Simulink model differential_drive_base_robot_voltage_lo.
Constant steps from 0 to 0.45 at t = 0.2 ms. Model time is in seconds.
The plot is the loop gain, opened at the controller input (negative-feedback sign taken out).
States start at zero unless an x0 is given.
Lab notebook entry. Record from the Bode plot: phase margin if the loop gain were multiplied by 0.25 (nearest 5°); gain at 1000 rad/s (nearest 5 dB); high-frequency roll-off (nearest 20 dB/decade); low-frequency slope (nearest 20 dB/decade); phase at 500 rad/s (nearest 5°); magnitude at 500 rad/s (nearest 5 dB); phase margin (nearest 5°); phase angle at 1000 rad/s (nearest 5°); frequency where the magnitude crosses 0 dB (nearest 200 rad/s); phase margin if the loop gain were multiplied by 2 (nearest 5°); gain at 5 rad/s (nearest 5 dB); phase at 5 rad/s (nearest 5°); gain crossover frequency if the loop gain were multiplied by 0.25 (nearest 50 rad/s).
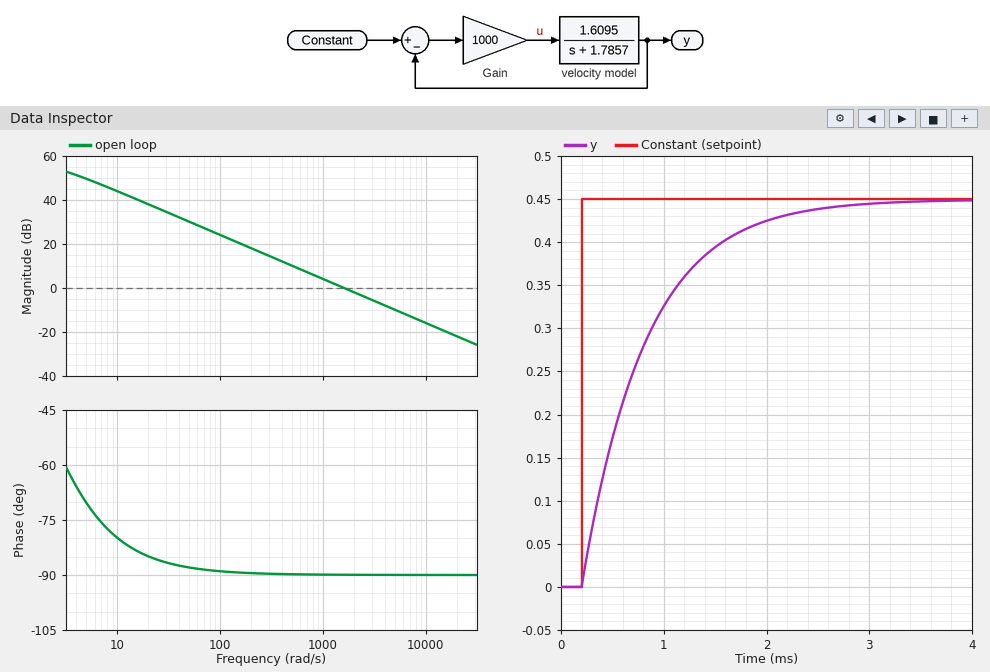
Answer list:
90°
5 dB
-20 dB/decade
-20 dB/decade
-90°
10 dB
90°
-90°
1600 rad/s
90°
50 dB
-70°
400 rad/s
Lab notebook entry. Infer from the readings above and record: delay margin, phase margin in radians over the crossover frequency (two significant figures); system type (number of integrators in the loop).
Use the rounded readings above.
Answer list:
0.00098 s
1
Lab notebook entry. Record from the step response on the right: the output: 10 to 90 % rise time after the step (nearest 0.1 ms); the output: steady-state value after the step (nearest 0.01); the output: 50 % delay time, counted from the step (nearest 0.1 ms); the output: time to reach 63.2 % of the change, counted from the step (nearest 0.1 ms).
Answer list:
1.4 ms
0.45
0.4 ms
0.6 ms
